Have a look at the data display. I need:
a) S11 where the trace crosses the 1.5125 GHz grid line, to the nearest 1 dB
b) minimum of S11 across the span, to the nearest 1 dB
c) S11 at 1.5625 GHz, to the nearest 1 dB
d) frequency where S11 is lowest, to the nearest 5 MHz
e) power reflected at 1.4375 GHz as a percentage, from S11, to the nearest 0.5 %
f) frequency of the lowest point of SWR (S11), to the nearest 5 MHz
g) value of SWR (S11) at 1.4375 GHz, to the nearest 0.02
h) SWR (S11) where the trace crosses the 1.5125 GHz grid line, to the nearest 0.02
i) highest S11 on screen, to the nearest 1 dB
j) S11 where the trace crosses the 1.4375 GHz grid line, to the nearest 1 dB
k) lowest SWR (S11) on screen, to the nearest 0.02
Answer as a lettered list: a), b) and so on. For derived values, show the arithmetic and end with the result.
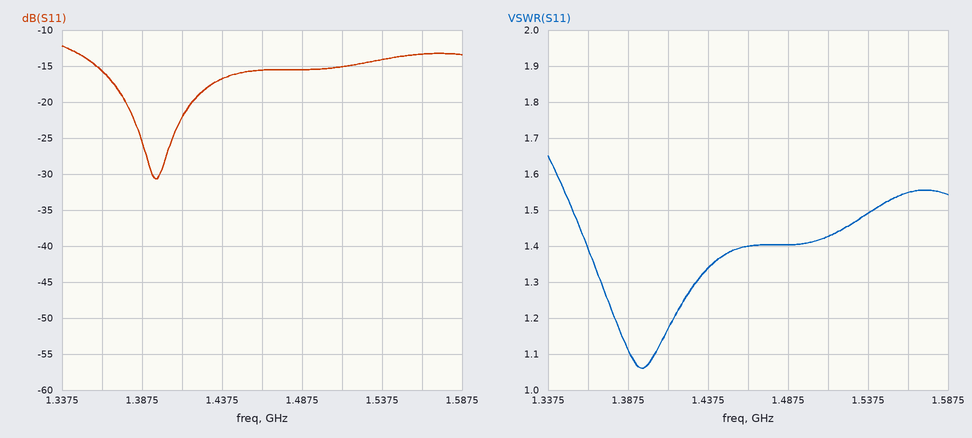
a) -15 dB
b) -31 dB
c) -13 dB
d) 1.395 GHz
e) 10^(-17/10) ≈ 2.0 %
f) 1.395 GHz
g) 1.34
h) 1.42
i) -12 dB
j) -17 dB
k) 1.06
